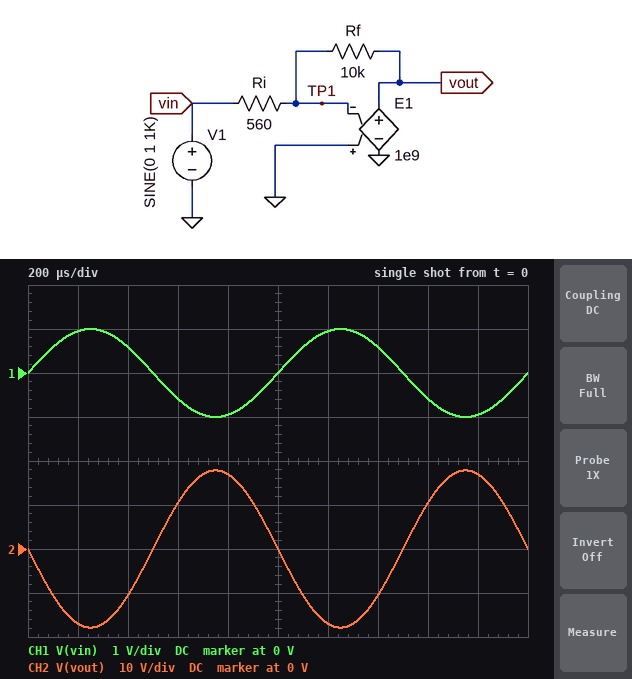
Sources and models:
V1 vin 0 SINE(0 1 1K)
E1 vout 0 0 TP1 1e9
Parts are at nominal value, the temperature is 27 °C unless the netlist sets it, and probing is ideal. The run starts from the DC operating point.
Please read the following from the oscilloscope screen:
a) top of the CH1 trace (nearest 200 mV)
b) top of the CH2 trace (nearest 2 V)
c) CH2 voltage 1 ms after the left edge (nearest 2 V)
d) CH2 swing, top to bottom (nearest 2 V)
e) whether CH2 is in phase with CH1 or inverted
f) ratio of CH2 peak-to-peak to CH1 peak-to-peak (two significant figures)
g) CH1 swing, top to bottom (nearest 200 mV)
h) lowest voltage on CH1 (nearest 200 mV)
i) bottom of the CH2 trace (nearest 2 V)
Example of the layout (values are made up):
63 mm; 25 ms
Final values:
1.0 V; 18 V; 0 V; 36 V; inverted; 18; 2.0 V; -1.0 V; -18 V
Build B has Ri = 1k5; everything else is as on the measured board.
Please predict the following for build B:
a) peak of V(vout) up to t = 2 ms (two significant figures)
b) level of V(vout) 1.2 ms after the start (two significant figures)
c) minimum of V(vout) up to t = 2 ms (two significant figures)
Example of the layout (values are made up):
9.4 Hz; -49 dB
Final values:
6.7 V; -6.3 V; -6.7 V
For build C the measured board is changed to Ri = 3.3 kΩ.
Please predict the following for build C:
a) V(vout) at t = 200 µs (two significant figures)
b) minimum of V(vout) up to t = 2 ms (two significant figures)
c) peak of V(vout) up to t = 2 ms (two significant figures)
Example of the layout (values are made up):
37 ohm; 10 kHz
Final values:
-2.9 V; -3.0 V; 3.0 V
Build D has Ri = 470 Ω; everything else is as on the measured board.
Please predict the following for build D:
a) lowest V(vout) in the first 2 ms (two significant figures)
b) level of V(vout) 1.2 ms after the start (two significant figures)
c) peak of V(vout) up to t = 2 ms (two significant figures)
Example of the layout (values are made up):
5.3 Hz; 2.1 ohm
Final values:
-21 V; -20 V; 21 V
